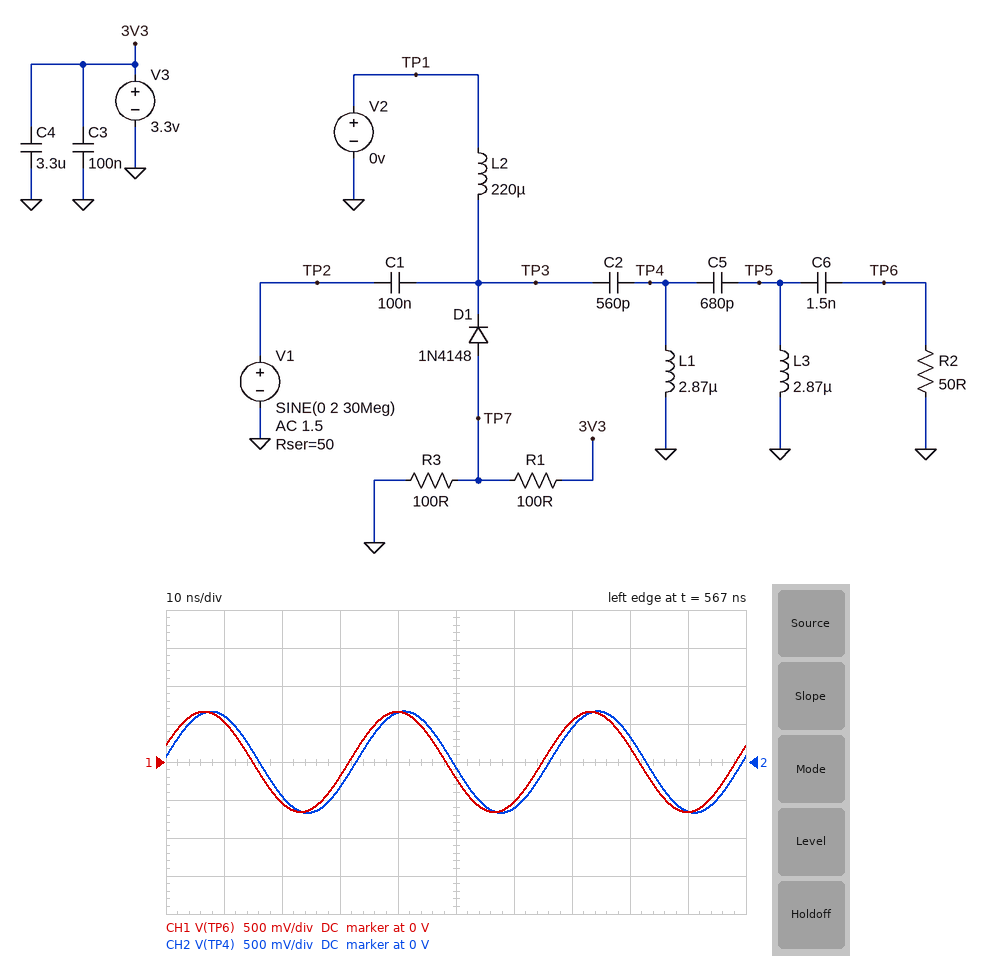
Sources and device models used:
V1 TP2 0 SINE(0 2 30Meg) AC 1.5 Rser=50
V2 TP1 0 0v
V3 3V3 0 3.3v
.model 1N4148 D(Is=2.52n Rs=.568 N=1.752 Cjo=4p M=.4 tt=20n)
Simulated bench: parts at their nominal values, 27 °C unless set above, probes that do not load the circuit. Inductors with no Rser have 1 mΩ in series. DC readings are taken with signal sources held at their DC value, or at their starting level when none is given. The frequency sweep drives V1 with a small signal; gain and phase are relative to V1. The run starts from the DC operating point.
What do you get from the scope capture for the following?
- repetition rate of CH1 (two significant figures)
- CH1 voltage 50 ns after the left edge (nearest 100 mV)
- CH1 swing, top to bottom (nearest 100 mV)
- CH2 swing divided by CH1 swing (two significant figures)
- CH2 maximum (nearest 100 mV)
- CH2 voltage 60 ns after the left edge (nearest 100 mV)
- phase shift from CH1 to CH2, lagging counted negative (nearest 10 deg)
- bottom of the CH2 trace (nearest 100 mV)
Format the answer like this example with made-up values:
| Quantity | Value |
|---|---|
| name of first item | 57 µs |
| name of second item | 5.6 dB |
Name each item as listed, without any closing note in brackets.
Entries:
| Quantity | Value |
|---|---|
| repetition rate of CH1 | 30 MHz |
| CH1 voltage 50 ns after the left edge | -200 mV |
| CH1 swing, top to bottom | 1.3 V |
| CH2 swing divided by CH1 swing | 1.0 |
| CH2 maximum | 700 mV |
| CH2 voltage 60 ns after the left edge | -600 mV |
| phase shift from CH1 to CH2, lagging counted negative | -10 deg |
| bottom of the CH2 trace | -700 mV |
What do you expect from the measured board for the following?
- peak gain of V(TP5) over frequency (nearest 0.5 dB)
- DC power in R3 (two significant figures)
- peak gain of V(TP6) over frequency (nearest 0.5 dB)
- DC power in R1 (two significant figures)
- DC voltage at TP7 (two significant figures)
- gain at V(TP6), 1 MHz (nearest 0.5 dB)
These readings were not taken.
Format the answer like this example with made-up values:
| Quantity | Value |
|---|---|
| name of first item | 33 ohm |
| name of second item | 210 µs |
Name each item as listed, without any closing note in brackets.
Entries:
| Quantity | Value |
|---|---|
| peak gain of V(TP5) over frequency | -9.0 dB |
| DC power in R3 | 5.3 mW |
| peak gain of V(TP6) over frequency | -9.5 dB |
| DC power in R1 | 66 mW |
| DC voltage at TP7 | 730 mV |
| gain at V(TP6), 1 MHz | -56.0 dB |
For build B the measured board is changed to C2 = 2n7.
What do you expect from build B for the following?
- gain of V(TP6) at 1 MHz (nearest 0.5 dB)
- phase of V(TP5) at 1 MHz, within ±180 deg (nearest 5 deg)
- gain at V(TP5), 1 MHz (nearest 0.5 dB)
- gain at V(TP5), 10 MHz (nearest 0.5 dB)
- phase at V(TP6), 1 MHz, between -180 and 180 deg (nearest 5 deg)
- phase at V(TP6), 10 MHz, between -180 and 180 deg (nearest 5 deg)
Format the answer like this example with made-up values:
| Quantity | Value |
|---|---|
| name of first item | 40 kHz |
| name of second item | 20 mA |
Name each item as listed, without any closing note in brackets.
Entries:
| Quantity | Value |
|---|---|
| gain of V(TP6) at 1 MHz | -41.0 dB |
| phase of V(TP5) at 1 MHz, within ±180 deg | -35 deg |
| gain at V(TP5), 1 MHz | -33.5 dB |
| gain at V(TP5), 10 MHz | -9.5 dB |
| phase at V(TP6), 1 MHz, between -180 and 180 deg | 30 deg |
| phase at V(TP6), 10 MHz, between -180 and 180 deg | 40 deg |
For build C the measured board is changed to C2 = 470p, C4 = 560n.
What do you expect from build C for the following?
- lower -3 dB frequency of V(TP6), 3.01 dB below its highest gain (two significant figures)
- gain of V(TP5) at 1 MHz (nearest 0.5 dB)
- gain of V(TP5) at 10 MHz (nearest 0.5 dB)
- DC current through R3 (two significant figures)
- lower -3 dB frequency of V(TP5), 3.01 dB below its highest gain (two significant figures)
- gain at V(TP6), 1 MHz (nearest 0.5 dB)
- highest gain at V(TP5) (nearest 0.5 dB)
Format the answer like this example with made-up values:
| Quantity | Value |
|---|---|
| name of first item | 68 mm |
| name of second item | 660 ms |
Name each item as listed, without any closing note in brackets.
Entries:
| Quantity | Value |
|---|---|
| lower -3 dB frequency of V(TP6), 3.01 dB below its highest gain | 2.7 MHz |
| gain of V(TP5) at 1 MHz | -50.0 dB |
| gain of V(TP5) at 10 MHz | -10.5 dB |
| DC current through R3 | 7.3 mA |
| lower -3 dB frequency of V(TP5), 3.01 dB below its highest gain | 2.1 MHz |
| gain at V(TP6), 1 MHz | -57.5 dB |
| highest gain at V(TP5) | -9.5 dB |
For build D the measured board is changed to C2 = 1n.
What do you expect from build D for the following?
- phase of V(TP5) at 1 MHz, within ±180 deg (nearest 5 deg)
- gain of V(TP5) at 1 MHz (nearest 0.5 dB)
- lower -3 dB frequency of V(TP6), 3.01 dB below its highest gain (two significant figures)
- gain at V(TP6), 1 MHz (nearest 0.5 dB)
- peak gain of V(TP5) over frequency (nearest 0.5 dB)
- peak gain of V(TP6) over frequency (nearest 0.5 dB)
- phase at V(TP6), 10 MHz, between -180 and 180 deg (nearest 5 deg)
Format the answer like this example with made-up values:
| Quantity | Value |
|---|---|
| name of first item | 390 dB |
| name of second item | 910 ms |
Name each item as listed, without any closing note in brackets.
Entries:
| Quantity | Value |
|---|---|
| phase of V(TP5) at 1 MHz, within ±180 deg | -15 deg |
| gain of V(TP5) at 1 MHz | -43.0 dB |
| lower -3 dB frequency of V(TP6), 3.01 dB below its highest gain | 1.9 MHz |
| gain at V(TP6), 1 MHz | -50.5 dB |
| peak gain of V(TP5) over frequency | -6.0 dB |
| peak gain of V(TP6) over frequency | -9.0 dB |
| phase at V(TP6), 10 MHz, between -180 and 180 deg | 45 deg |
